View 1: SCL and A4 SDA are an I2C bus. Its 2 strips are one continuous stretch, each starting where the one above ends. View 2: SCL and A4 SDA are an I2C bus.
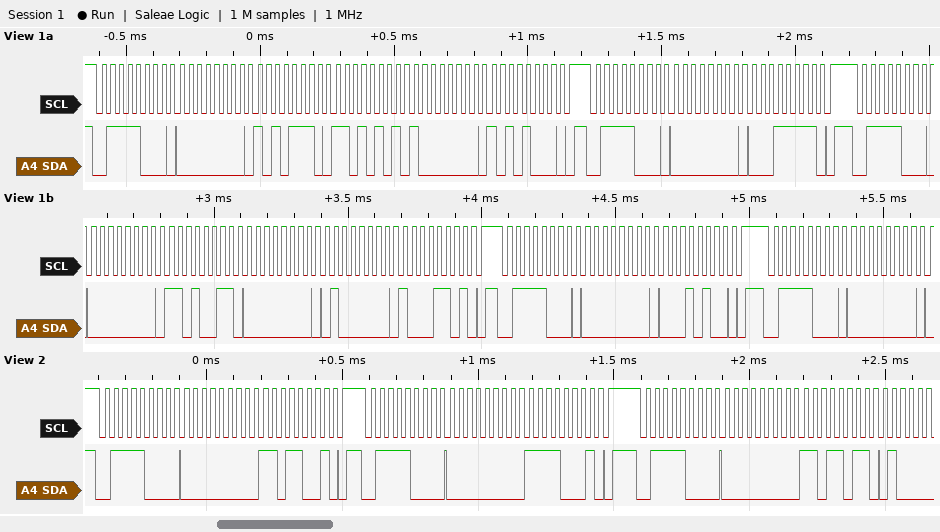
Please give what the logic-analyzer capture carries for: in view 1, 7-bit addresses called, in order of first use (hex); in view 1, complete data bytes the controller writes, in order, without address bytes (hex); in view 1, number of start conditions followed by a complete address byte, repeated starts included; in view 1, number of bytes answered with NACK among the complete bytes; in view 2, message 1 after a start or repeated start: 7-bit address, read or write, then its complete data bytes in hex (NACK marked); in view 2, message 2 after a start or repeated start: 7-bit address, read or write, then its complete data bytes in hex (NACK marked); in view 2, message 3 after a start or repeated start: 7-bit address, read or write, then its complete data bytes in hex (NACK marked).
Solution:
0x3C
00 AE D5 80 A8 00 1F 00 D3 00 40 8D 00 14 00
5
0
0x3C write: 00 D9
0x3C write: 00 F1
0x3C write: 00 DB
